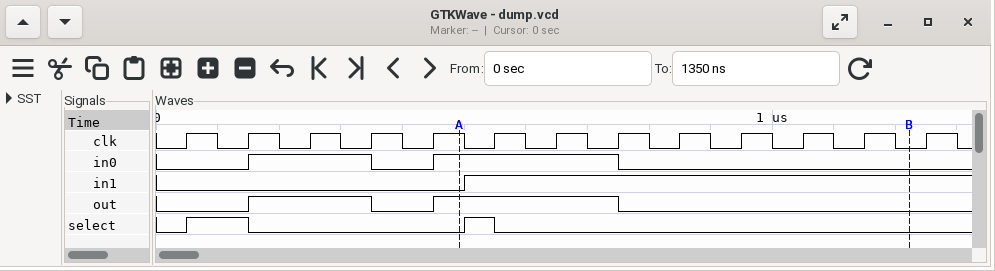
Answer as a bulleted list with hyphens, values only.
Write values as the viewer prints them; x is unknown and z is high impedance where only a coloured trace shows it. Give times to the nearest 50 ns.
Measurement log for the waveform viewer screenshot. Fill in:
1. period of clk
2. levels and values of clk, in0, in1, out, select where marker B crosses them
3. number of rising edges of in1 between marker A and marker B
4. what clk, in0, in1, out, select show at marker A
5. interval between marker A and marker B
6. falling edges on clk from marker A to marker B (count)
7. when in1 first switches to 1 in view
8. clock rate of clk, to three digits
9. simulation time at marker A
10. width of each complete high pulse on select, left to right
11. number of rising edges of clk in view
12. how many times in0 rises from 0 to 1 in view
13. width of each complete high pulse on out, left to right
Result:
- 100 ns
- clk=0, in0=0, in1=1, out=0, select=0
- 1
- clk=1, in0=1, in1=0, out=1, select=0
- 750 ns
- 8
- 500 ns
- 10.0 MHz
- 500 ns
- 100 ns, 50 ns
- 13
- 2
- 200 ns, 300 ns
